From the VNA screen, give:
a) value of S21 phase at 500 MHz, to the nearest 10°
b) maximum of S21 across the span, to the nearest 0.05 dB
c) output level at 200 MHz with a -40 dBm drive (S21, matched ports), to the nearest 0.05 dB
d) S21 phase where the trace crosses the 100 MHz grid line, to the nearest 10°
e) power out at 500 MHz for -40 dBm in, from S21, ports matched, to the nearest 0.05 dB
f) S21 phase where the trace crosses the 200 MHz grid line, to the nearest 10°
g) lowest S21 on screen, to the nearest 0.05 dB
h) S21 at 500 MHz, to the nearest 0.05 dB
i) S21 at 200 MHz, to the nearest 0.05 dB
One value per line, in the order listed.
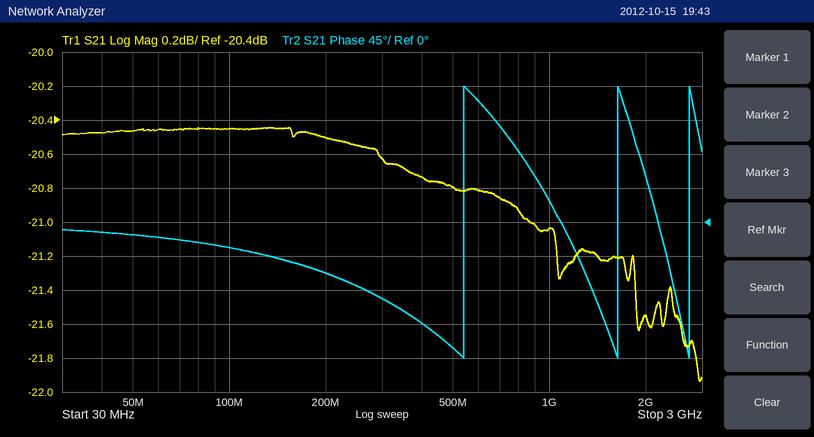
-170°
-20.45 dB
-60.50 dBm
-30°
-60.80 dBm
-70°
-21.95 dB
-20.80 dB
-20.50 dB
